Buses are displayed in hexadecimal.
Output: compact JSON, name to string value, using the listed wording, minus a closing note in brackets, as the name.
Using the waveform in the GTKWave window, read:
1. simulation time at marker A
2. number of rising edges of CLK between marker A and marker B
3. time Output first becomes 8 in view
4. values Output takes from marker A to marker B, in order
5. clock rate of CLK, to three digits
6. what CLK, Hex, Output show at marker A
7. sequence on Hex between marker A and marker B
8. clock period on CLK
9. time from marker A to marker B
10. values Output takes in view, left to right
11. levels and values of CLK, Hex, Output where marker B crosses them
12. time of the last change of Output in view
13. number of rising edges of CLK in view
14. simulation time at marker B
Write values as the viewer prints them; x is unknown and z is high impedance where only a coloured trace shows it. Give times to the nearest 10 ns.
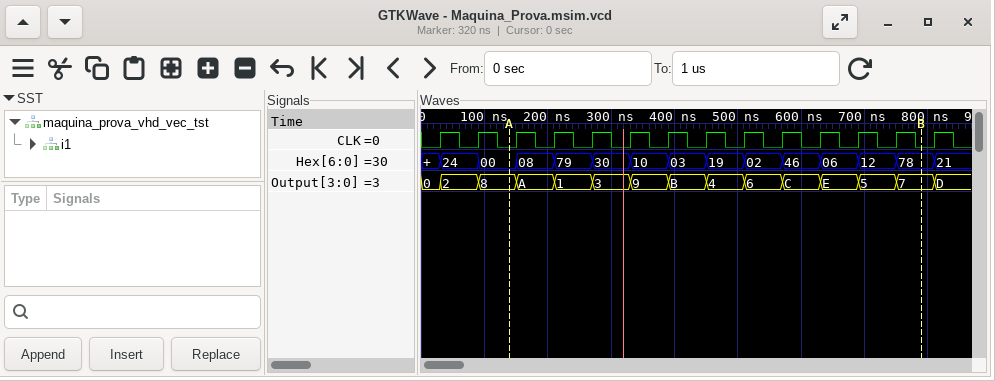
{"simulation time at marker A": "140 ns", "number of rising edges of CLK between marker A and marker B": "11", "time Output first becomes 8 in view": "90 ns", "values Output takes from marker A to marker B, in order": "8, A, 1, 3, 9, B, 4, 6, C, E, 5, 7", "clock rate of CLK, to three digits": "16.7 MHz", "what CLK, Hex, Output show at marker A": "CLK=0, Hex=00, Output=8", "sequence on Hex between marker A and marker B": "00, 08, 79, 30, 10, 03, 19, 02, 46, 06, 12, 78", "clock period on CLK": "60 ns", "time from marker A to marker B": "650 ns", "values Output takes in view, left to right": "0, 2, 8, A, 1, 3, 9, B, 4, 6, C, E, 5, 7, D", "levels and values of CLK, Hex, Output where marker B crosses them": "CLK=0, Hex=78, Output=7", "time of the last change of Output in view": "810 ns", "number of rising edges of CLK in view": "14", "simulation time at marker B": "790 ns"}
